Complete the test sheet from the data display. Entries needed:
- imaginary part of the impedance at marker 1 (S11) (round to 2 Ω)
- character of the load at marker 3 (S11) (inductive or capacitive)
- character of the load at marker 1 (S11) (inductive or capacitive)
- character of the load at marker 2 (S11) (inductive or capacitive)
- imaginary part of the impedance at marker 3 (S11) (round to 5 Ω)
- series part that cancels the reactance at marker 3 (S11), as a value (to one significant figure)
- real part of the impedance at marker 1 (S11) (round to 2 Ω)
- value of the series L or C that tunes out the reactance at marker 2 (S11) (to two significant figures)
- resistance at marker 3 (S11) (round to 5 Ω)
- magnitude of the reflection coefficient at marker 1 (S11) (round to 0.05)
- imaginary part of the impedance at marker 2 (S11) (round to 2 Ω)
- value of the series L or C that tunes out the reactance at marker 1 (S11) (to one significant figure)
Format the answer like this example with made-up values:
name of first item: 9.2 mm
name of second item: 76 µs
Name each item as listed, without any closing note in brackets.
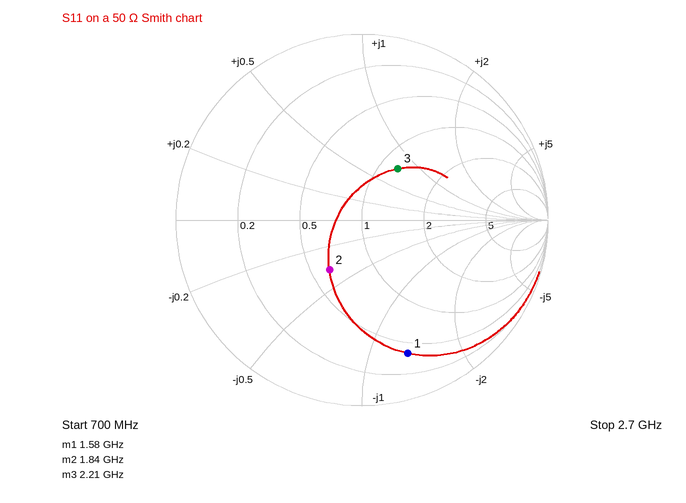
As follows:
imaginary part of the impedance at marker 1 (S11): -66 Ω
character of the load at marker 3 (S11): inductive
character of the load at marker 1 (S11): capacitive
character of the load at marker 2 (S11): capacitive
imaginary part of the impedance at marker 3 (S11): +40 Ω
series part that cancels the reactance at marker 3 (S11), as a value: 2 pF
real part of the impedance at marker 1 (S11): 20 Ω
value of the series L or C that tunes out the reactance at marker 2 (S11): 1.6 nH
resistance at marker 3 (S11): 60 Ω
magnitude of the reflection coefficient at marker 1 (S11): 0.75
imaginary part of the impedance at marker 2 (S11): -18 Ω
value of the series L or C that tunes out the reactance at marker 1 (S11): 7 nH
